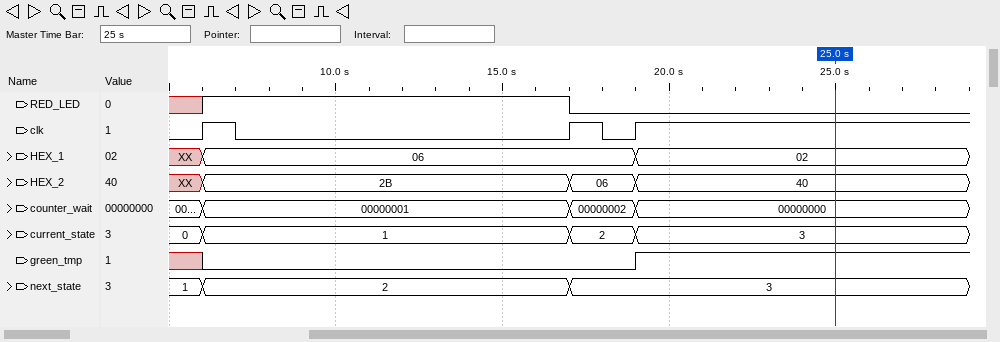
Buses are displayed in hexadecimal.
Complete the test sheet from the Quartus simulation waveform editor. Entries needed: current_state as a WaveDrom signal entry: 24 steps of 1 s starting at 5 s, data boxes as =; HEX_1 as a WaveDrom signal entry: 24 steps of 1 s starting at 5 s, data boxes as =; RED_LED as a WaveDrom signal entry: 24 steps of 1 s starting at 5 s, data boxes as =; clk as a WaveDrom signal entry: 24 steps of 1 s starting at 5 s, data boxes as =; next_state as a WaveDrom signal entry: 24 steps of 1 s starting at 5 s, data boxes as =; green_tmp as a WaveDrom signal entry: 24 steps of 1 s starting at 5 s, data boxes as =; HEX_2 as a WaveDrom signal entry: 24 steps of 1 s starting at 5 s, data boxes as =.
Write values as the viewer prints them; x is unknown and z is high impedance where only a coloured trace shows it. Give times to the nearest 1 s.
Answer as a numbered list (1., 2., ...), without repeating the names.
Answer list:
1. {name: 'current_state', wave: '==..........=.=.........', data: '0 1 2 3'}
2. {name: 'HEX_1', wave: 'x=............=.........', data: '06 02'}
3. {name: 'RED_LED', wave: 'x1..........0...........'}
4. {name: 'clk', wave: '010.........101.........'}
5. {name: 'next_state', wave: '==..........=...........', data: '1 2 3'}
6. {name: 'green_tmp', wave: 'x0............1.........'}
7. {name: 'HEX_2', wave: 'x=..........=.=.........', data: '2B 06 40'}
